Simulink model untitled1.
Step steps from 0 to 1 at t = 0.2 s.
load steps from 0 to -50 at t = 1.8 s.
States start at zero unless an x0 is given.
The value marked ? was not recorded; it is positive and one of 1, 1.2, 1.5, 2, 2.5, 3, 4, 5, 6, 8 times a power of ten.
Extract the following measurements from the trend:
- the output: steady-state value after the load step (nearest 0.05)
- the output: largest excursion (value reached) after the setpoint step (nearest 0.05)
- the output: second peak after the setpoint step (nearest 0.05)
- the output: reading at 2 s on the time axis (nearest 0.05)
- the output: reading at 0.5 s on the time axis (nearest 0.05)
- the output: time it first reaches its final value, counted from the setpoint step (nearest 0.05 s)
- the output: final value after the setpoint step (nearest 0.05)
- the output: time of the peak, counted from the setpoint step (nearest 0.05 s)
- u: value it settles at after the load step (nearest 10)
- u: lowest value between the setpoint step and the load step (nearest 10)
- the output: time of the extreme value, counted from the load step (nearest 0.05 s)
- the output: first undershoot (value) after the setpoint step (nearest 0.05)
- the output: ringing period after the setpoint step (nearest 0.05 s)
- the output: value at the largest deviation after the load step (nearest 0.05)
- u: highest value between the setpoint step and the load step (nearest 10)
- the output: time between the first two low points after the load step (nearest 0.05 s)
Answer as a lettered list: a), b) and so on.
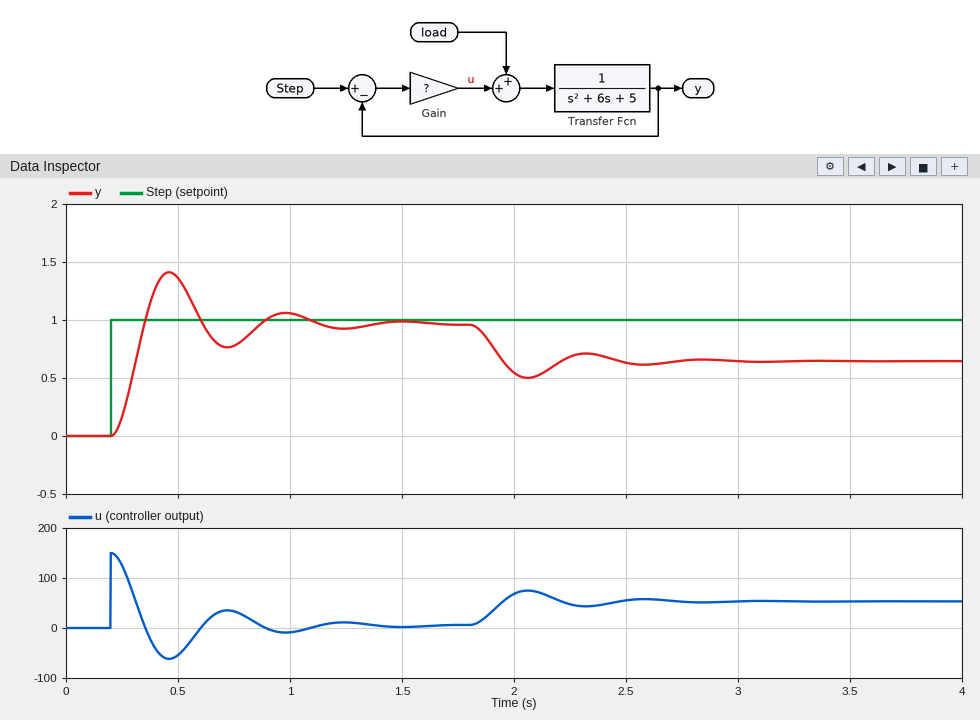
a) 0.65
b) 1.40
c) 1.05
d) 0.55
e) 1.35
f) 0.15 s
g) 0.95
h) 0.25 s
i) 50
j) -60
k) 0.25 s
l) 0.75
m) 0.50 s
n) 0.50
o) 150
p) 0.50 s
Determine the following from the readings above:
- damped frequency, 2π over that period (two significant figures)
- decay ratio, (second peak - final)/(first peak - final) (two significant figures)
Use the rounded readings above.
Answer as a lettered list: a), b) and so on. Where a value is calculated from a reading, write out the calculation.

a) 2π / 0.5 = 13 rad/s
b) (1.05 - 0.95) / (1.4 - 0.95) = 0.22
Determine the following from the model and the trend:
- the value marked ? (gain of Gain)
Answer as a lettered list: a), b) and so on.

a) 150
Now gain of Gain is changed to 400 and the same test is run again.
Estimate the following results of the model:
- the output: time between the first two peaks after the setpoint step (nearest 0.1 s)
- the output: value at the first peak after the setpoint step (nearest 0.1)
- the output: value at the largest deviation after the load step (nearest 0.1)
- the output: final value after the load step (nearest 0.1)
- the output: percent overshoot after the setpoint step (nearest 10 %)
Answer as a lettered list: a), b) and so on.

a) 0.3 s
b) 1.6
c) 0.8
d) 0.9
e) 60 %
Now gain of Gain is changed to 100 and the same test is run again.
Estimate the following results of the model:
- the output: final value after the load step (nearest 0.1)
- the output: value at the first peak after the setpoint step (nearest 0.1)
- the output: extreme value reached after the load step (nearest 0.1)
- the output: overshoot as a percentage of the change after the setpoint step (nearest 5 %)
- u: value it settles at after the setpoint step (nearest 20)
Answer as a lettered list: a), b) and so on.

a) 0.5
b) 1.3
c) 0.3
d) 40 %
e) 0
